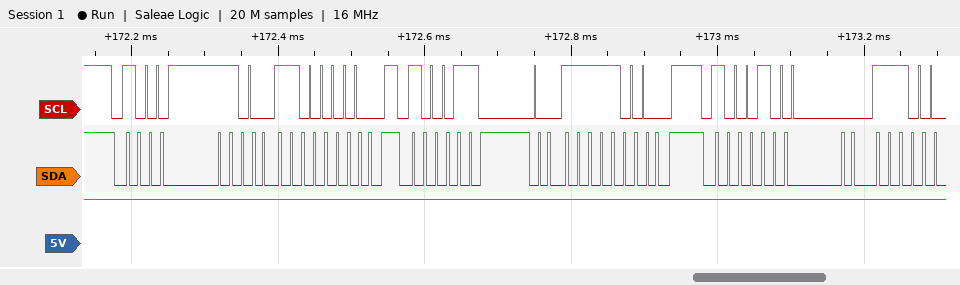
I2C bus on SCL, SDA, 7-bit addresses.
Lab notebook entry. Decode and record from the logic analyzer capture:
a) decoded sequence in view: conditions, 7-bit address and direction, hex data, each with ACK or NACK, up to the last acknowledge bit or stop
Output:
start, address 46 write ACK, C0 ACK, stop, start, address 46 write ACK, F8 ACK, stop, start, address 44 write ACK
